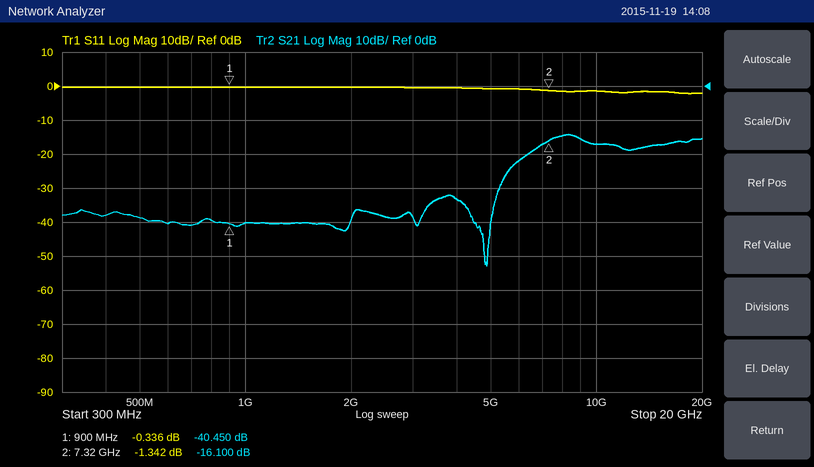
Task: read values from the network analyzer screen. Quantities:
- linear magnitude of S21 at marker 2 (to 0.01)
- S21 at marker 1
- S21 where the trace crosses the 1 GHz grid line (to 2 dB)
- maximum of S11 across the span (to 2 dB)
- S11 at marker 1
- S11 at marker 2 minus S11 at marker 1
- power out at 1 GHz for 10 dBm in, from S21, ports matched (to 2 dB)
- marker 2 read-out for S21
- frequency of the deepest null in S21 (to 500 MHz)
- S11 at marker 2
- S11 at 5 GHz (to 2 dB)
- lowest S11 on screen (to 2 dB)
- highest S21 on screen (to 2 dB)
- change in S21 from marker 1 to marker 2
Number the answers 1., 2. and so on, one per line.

1. 0.16
2. -40.450 dB
3. -40 dB
4. 0 dB
5. -0.336 dB
6. -1.006 dB
7. -30 dBm
8. -16.100 dB
9. 5.0 GHz
10. -1.342 dB
11. 0 dB
12. -2 dB
13. -14 dB
14. 24.350 dB
